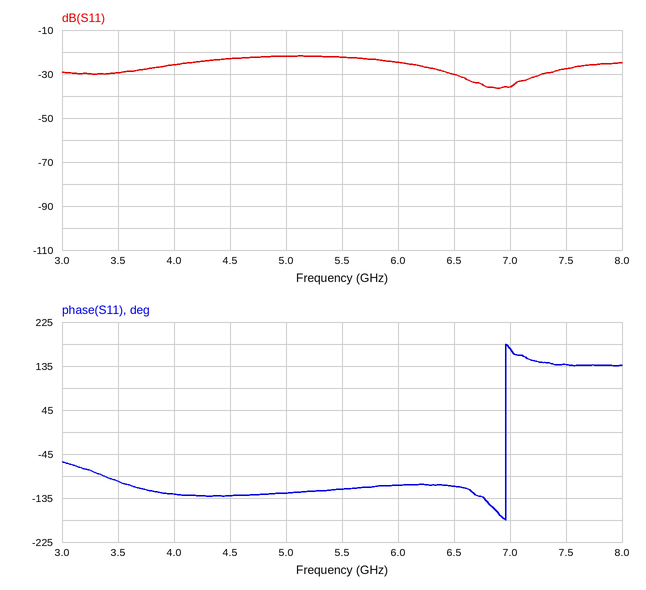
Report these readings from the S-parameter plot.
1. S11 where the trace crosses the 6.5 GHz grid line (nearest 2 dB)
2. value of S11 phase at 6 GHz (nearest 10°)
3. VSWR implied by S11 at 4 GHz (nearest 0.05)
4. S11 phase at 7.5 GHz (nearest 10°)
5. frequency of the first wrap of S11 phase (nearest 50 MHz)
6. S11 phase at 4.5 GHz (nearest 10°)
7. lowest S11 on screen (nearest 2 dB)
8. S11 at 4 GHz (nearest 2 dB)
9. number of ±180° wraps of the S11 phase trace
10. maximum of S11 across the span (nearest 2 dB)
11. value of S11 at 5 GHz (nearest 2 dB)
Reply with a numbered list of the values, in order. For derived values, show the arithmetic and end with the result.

1. -30 dB
2. -110°
3. |Γ| = 10^(-26/20) = 0.0501; VSWR = (1 + 0.0501)/(1 − 0.0501) ≈ 1.11, so 1.10 to the nearest 0.05
4. 140°
5. 6.95 GHz
6. -130°
7. -36 dB
8. -26 dB
9. 1
10. -22 dB
11. -22 dB
